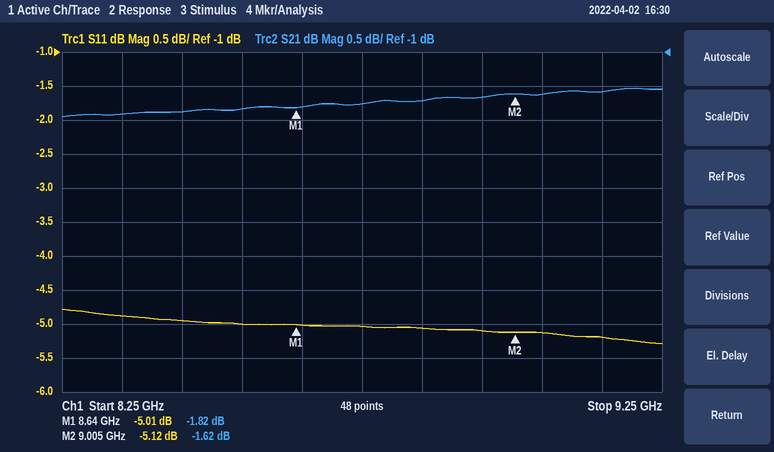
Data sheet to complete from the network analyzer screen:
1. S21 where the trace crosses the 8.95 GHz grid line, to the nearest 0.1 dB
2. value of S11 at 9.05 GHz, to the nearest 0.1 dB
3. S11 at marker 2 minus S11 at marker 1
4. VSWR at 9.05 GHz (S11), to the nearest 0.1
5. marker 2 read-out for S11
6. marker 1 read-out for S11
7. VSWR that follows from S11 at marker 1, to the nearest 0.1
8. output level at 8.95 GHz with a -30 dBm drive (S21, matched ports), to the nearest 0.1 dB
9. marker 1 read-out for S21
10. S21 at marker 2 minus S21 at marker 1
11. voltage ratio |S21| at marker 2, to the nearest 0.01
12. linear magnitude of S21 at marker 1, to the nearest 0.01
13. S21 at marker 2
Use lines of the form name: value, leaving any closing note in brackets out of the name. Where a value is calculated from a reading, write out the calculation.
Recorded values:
S21 where the trace crosses the 8.95 GHz grid line, to the nearest 0.1 dB: -1.7 dB
value of S11 at 9.05 GHz, to the nearest 0.1 dB: -5.1 dB
S11 at marker 2 minus S11 at marker 1: -5.12 − (-5.01) = -0.11 dB
VSWR at 9.05 GHz (S11), to the nearest 0.1: |Γ| = 10^(-5.1/20) = 0.5559; VSWR = (1 + 0.5559)/(1 − 0.5559) ≈ 3.5
marker 2 read-out for S11: -5.12 dB
marker 1 read-out for S11: -5.01 dB
VSWR that follows from S11 at marker 1, to the nearest 0.1: (1 + 0.5617)/(1 − 0.5617) ≈ 3.6
output level at 8.95 GHz with a -30 dBm drive (S21, matched ports), to the nearest 0.1 dB: -30 dBm + (-1.7 dB) = -31.7 dBm
marker 1 read-out for S21: -1.82 dB
S21 at marker 2 minus S21 at marker 1: -1.62 − (-1.82) = 0.20 dB
voltage ratio |S21| at marker 2, to the nearest 0.01: 10^(-1.62/20) ≈ 0.83
linear magnitude of S21 at marker 1, to the nearest 0.01: 10^(-1.82/20) ≈ 0.81
S21 at marker 2: -1.62 dB
